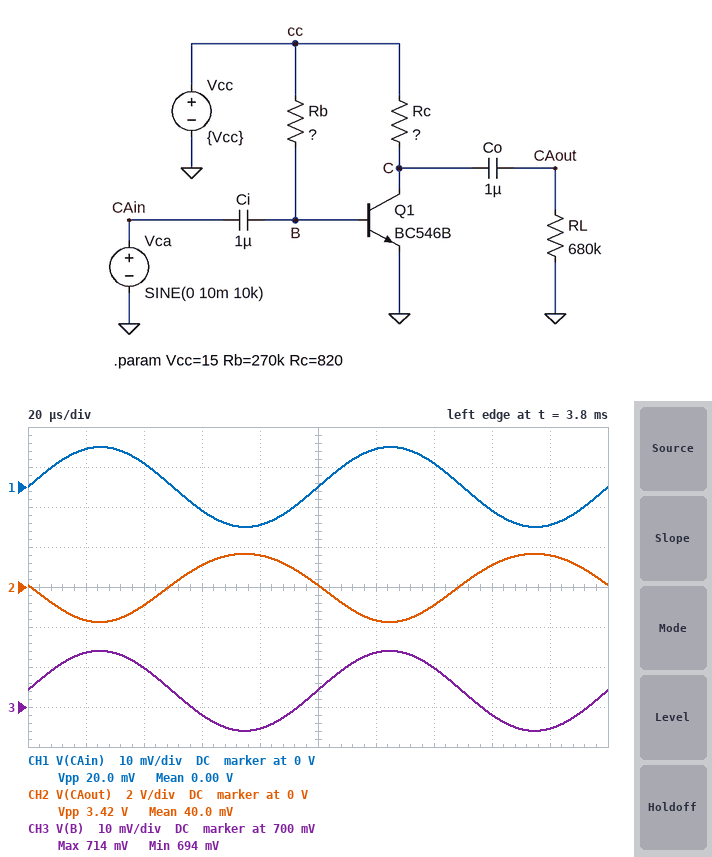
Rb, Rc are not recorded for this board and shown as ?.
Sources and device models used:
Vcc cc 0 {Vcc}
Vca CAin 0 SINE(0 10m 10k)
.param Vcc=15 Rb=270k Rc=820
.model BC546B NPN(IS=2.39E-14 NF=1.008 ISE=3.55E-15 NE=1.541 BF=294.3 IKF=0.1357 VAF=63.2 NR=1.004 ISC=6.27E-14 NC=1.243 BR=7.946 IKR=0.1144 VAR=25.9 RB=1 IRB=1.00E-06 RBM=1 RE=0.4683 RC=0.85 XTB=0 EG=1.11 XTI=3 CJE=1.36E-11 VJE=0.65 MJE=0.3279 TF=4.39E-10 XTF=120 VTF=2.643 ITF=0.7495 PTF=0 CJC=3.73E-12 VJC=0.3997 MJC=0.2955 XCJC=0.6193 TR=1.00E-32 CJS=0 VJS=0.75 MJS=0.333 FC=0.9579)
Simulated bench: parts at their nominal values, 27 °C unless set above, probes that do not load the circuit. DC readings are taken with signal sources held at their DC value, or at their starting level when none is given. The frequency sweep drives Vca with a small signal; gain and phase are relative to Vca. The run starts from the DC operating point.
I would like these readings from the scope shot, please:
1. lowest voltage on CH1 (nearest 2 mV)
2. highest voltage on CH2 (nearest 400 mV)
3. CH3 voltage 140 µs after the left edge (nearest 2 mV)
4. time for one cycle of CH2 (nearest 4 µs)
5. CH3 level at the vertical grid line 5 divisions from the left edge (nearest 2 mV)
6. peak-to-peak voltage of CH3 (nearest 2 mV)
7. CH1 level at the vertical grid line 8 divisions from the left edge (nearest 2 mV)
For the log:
-10 mV
1.6 V
710 mV
100 µs
704 mV
20 mV
-6 mV
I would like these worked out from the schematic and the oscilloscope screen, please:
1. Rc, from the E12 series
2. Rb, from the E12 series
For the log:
560 Ω
390 kΩ
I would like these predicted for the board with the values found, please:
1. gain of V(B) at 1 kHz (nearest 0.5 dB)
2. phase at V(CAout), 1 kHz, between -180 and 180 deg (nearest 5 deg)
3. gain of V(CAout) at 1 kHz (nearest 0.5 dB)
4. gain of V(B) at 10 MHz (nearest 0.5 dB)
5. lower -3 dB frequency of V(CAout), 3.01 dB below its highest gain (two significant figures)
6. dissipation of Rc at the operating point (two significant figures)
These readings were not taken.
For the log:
0 dB
-170 deg
44.5 dB
0 dB
190 Hz
68 mW
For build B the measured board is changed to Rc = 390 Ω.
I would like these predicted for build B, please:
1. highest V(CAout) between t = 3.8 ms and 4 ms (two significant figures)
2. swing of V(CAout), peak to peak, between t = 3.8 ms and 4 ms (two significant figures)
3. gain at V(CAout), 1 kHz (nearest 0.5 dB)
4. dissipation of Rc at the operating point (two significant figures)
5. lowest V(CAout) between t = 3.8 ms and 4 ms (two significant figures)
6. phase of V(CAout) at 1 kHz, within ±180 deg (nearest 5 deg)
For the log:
1.2 V
2.5 V
42.0 dB
50 mW
-1.3 V
-170 deg
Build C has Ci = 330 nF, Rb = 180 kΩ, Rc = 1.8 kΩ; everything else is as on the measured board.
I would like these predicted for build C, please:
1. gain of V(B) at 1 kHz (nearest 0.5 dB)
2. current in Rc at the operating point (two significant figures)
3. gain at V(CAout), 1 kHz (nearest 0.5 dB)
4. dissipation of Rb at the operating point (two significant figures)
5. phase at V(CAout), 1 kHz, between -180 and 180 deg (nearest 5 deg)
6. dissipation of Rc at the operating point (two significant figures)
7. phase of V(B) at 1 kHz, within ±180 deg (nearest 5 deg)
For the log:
-25.5 dB
8.3 mA
1.0 dB
1.1 mW
-95 deg
120 mW
85 deg
